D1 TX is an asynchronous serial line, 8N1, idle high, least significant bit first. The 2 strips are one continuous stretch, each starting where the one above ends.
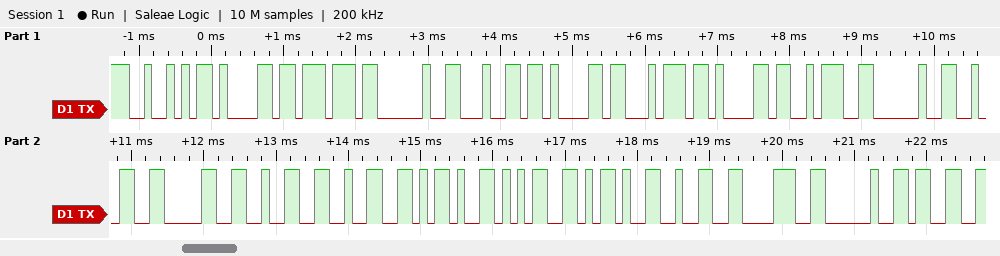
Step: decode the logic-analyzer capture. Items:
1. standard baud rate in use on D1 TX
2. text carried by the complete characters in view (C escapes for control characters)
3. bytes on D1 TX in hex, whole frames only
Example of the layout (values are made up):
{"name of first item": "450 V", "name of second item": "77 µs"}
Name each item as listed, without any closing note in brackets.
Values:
{"standard baud rate in use on D1 TX": "9600 baud", "text carried by the complete characters in view": "\"Raw data: 2022-5-28 3\"", "bytes on D1 TX in hex, whole frames only": "0x52 0x61 0x77 0x20 0x64 0x61 0x74 0x61 0x3A 0x20 0x32 0x30 0x32 0x32 0x2D 0x35 0x2D 0x32 0x38 0x20 0x33"}
